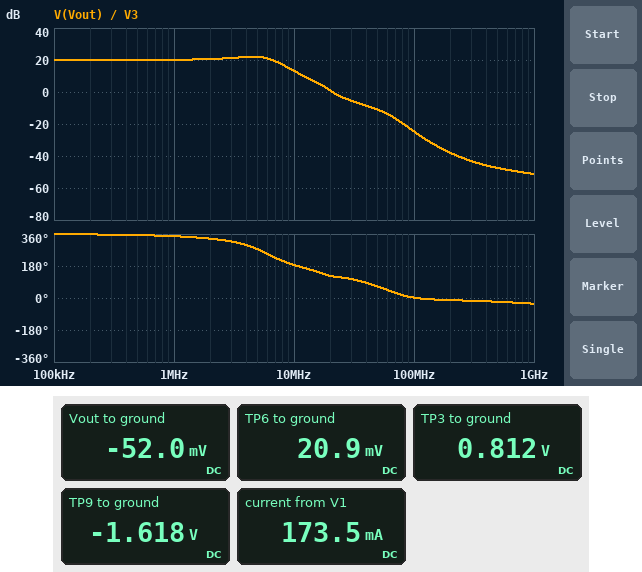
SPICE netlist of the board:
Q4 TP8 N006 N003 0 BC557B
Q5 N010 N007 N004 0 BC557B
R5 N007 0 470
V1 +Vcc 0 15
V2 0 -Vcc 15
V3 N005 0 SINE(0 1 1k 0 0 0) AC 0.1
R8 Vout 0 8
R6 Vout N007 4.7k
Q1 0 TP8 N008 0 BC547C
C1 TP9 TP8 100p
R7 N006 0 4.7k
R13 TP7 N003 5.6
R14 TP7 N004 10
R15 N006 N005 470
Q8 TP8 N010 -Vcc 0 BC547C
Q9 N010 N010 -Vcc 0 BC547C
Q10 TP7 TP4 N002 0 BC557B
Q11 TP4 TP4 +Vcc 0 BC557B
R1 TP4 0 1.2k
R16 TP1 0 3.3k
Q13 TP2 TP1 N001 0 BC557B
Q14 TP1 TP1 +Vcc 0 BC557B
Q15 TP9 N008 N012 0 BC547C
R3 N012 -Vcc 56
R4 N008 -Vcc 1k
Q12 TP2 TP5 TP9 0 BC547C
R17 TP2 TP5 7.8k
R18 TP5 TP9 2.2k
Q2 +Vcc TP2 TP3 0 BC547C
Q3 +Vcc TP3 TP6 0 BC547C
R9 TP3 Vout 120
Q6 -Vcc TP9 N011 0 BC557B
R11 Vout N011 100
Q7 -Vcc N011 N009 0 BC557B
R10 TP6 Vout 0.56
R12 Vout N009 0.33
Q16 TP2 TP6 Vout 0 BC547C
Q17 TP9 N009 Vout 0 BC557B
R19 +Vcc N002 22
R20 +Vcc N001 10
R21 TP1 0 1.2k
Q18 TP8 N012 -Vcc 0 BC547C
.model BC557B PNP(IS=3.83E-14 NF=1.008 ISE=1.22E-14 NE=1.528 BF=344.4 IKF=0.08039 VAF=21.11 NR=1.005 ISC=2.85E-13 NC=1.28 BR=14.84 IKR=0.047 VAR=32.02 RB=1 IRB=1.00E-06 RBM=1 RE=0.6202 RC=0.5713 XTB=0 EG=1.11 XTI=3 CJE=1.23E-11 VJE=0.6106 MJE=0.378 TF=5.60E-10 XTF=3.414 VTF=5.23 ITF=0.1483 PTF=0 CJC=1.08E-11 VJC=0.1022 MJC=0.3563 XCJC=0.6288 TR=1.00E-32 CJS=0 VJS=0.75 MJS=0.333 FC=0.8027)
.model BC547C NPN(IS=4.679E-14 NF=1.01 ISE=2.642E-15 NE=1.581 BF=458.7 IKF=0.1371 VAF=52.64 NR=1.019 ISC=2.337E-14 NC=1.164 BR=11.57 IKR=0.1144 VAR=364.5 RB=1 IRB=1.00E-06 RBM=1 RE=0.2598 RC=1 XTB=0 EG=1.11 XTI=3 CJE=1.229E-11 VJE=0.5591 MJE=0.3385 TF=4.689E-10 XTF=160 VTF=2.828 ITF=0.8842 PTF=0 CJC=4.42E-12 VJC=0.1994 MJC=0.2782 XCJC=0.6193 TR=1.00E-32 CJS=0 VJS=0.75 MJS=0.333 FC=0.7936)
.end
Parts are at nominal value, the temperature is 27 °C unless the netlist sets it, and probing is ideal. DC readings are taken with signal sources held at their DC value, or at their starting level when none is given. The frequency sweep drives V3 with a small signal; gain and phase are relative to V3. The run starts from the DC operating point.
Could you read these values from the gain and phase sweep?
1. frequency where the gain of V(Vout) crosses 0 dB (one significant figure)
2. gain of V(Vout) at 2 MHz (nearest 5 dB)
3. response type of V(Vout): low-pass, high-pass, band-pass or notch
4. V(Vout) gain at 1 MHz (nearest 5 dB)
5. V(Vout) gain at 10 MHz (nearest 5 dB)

20 MHz
20 dB
low-pass
20 dB
15 dB
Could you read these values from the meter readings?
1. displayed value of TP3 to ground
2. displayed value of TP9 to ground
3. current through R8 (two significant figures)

0.812 V
-1.618 V
6.5 mA
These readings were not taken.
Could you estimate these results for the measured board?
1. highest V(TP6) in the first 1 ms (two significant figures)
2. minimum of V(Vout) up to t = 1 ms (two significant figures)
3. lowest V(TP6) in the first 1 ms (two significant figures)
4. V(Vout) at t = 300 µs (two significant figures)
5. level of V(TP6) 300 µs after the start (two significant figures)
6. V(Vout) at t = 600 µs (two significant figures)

10 V
-10 V
-10 V
9.5 V
10 V
-5.9 V
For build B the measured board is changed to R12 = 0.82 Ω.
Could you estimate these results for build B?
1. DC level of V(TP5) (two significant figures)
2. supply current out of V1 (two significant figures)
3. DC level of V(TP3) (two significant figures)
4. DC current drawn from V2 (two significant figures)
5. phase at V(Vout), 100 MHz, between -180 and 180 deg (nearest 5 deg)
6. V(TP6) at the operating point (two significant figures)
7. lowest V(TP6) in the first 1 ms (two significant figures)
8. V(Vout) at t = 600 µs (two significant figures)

-980 mV
150 mA
790 mV
130 mA
5 deg
8.4 mV
-6.8 V
-5.9 V
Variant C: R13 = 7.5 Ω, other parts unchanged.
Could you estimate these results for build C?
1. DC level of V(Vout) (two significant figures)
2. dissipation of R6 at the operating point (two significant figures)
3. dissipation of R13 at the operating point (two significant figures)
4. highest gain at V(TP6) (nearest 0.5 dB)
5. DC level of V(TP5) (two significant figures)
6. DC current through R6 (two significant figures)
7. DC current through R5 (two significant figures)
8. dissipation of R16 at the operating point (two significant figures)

-23 mV
100 nW
14 µW
22.0 dB
-920 mV
4.7 µA
2.2 µA
62 mW
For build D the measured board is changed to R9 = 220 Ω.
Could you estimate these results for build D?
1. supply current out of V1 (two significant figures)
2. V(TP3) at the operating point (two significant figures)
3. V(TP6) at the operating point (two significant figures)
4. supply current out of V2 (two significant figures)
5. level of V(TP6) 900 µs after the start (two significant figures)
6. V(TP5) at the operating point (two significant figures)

180 mA
820 mV
26 mV
160 mA
-5.9 V
-960 mV
